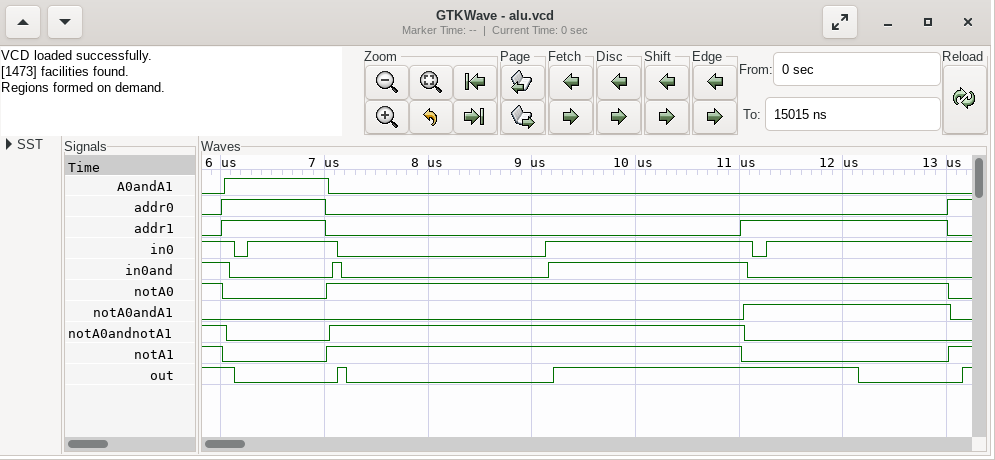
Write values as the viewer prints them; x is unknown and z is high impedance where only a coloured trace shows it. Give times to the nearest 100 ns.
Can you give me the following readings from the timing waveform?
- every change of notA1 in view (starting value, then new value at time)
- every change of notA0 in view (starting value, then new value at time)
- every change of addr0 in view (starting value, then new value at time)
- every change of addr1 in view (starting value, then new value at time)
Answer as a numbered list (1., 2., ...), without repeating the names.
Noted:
1. 1, 0 at 6000 ns, 1 at 7000 ns, 0 at 11000 ns, 1 at 13000 ns
2. 1, 0 at 6000 ns, 1 at 7000 ns, 0 at 13000 ns
3. 0, 1 at 6000 ns, 0 at 7000 ns, 1 at 13000 ns
4. 0, 1 at 6000 ns, 0 at 7000 ns, 1 at 11000 ns, 0 at 13000 ns
